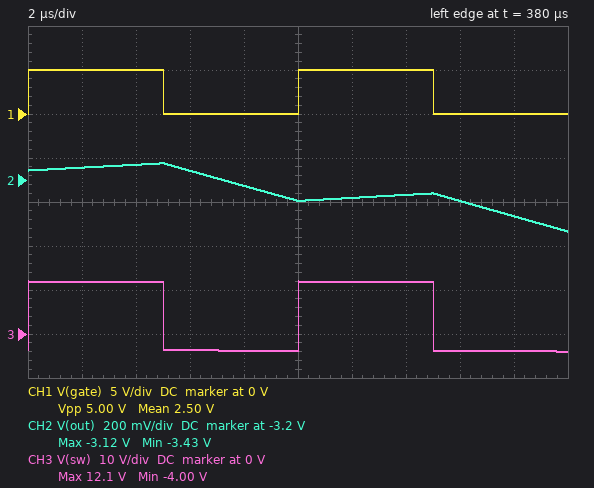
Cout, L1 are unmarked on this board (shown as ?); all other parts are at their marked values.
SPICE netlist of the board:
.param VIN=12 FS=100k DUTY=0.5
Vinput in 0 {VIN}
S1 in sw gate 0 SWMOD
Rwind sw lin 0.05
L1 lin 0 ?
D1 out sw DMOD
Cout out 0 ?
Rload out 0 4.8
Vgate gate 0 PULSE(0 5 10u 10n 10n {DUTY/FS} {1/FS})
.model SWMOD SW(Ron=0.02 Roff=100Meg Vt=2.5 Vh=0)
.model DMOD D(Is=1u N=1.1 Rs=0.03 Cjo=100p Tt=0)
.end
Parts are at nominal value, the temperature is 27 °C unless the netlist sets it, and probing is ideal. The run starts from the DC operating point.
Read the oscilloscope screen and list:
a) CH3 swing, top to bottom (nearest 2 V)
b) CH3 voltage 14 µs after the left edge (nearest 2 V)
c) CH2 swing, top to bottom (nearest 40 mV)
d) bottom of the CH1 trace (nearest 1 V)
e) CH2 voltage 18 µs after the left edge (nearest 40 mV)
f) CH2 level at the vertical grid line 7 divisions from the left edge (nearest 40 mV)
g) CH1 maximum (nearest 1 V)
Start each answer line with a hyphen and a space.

- 16 V
- 12 V
- 320 mV
- 0 V
- -3.36 V
- -3.28 V
- 5 V
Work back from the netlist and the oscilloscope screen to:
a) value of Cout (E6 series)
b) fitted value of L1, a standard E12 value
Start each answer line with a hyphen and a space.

- 100 µF
- 470 µH
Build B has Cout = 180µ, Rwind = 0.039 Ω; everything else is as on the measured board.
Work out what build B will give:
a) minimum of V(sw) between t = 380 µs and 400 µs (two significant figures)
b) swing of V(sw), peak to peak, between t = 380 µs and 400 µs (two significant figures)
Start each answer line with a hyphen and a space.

- -2.8 V
- 15 V
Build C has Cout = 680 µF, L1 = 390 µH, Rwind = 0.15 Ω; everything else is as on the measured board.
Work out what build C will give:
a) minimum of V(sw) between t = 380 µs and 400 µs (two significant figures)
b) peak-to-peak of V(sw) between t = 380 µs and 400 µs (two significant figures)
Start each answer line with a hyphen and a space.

- -1.4 V
- 13 V
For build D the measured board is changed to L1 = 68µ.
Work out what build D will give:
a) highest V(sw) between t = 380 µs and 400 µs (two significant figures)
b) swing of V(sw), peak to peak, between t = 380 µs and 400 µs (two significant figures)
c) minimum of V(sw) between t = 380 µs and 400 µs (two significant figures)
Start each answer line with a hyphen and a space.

- 12 V
- 27 V
- -15 V
